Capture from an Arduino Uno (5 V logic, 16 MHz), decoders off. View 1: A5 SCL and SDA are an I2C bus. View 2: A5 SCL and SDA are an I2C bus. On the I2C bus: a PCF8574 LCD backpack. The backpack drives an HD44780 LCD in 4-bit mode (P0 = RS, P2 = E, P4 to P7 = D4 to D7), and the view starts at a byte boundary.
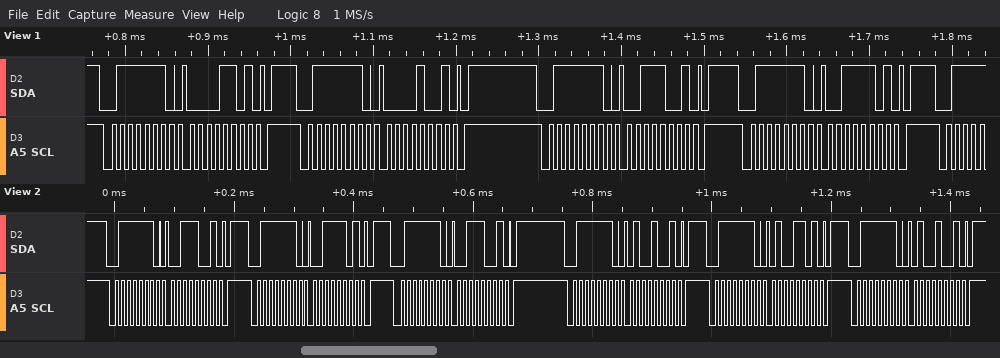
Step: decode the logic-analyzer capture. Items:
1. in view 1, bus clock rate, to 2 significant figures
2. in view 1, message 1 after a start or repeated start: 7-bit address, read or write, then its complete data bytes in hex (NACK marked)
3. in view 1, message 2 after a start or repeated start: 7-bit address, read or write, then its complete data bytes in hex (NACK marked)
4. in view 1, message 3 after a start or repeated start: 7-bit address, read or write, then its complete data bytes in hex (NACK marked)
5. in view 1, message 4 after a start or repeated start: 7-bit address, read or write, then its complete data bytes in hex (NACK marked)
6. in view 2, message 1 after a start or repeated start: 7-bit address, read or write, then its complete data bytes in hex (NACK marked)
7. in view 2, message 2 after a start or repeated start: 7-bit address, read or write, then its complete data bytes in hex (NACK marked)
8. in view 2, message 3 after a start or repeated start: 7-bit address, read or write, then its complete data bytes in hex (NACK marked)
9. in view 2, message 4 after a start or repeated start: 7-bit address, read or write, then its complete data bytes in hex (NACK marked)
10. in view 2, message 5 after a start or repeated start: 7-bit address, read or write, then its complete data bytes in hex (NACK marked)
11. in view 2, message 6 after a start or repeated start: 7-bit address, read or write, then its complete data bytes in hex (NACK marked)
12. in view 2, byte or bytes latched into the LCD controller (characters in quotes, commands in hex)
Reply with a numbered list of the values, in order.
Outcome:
1. 100 kHz
2. 0x3F write: 0D
3. 0x3F write: 09
4. 0x3F write: 39
5. 0x3F write: 3D
6. 0x3F write: 39
7. 0x3F write: 3D
8. 0x3F write: 39
9. 0x3F write: 49
10. 0x3F write: 4D
11. 0x3F write: 49
12. '4'
